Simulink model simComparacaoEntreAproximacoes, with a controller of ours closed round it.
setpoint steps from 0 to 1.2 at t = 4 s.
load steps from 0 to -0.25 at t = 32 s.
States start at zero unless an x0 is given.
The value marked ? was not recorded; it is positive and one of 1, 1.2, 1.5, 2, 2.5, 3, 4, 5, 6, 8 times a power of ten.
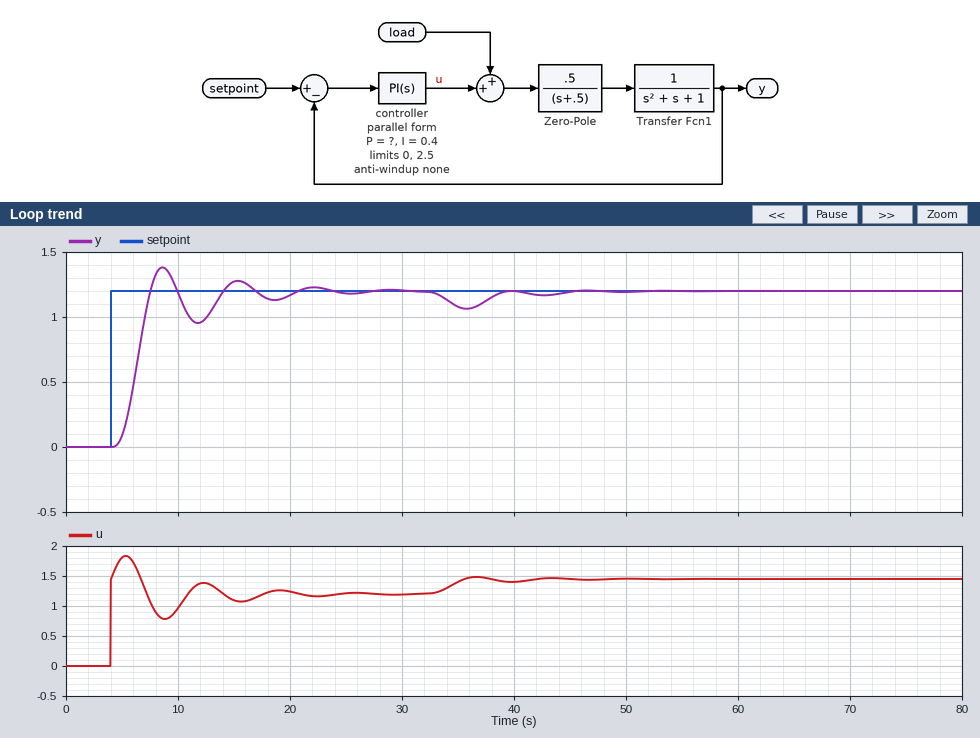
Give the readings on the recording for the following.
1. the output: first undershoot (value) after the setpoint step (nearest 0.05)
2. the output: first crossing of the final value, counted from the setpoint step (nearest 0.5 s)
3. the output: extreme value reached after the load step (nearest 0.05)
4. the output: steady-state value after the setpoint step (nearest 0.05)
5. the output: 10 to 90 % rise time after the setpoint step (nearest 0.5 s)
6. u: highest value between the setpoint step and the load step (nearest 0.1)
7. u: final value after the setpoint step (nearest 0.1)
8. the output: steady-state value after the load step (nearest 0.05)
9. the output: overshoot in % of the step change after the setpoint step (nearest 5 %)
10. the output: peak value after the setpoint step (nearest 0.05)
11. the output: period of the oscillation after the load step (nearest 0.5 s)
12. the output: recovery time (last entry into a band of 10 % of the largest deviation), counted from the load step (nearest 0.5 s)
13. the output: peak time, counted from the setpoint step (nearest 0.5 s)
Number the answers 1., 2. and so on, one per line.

1. 0.95
2. 3.5 s
3. 1.05
4. 1.20
5. 2.0 s
6. 1.8
7. 1.2
8. 1.20
9. 15 %
10. 1.40
11. 7.0 s
12. 12.5 s
13. 4.5 s
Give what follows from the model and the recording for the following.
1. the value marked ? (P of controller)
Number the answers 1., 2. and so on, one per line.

1. 1.2
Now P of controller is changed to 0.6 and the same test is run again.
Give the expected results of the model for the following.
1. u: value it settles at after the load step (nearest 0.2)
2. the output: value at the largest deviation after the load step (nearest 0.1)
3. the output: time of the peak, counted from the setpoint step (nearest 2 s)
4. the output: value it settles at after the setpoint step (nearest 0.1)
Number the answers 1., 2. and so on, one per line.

1. 1.4
2. 1.0
3. 6 s
4. 1.2
